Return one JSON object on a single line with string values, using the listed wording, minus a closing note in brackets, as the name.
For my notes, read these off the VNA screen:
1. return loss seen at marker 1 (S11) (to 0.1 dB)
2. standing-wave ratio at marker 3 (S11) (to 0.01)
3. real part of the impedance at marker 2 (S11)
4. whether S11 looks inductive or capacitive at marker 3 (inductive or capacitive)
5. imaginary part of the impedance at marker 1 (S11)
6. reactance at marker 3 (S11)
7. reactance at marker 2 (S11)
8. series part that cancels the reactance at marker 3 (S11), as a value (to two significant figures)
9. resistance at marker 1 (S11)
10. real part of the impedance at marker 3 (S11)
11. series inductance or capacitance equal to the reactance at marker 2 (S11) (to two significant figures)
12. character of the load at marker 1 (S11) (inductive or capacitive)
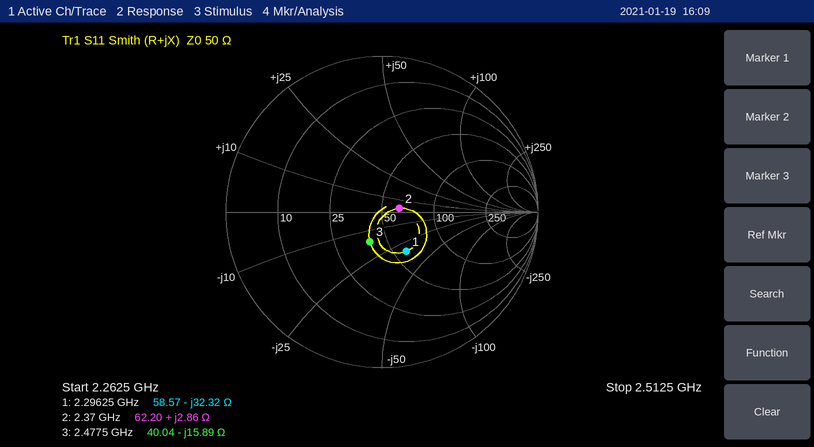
{"return loss seen at marker 1 (S11)": "10.6 dB", "standing-wave ratio at marker 3 (S11)": "1.52", "real part of the impedance at marker 2": "62.20 Ω", "whether S11 looks inductive or capacitive at marker 3": "capacitive", "imaginary part of the impedance at marker 1": "-32.32 Ω", "reactance at marker 3": "-15.89 Ω", "reactance at marker 2": "+2.86 Ω", "series part that cancels the reactance at marker 3 (S11), as a value": "1.0 nH", "resistance at marker 1": "58.57 Ω", "real part of the impedance at marker 3": "40.04 Ω", "series inductance or capacitance equal to the reactance at marker 2 (S11)": "190 pH", "character of the load at marker 1 (S11)": "capacitive"}
